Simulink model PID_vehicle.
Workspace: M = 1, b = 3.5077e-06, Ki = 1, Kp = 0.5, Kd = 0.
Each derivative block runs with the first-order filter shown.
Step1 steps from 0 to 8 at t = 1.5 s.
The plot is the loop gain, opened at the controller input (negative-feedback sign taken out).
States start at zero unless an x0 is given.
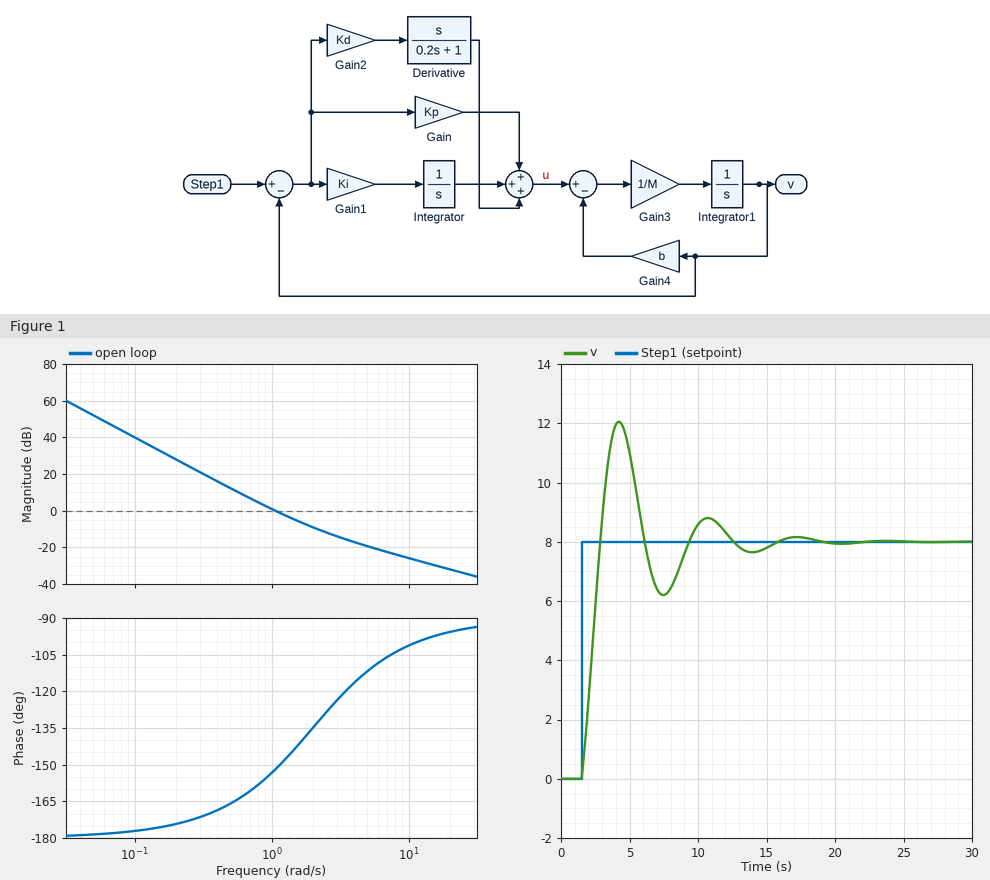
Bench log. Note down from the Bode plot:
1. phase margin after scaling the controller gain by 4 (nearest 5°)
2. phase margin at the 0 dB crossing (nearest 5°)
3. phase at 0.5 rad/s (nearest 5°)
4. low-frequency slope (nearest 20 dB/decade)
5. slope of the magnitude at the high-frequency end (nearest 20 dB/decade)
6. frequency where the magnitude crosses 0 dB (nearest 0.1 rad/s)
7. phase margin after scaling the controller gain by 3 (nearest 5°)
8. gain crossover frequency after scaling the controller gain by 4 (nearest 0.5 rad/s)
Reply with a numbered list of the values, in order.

1. 50°
2. 30°
3. -165°
4. -40 dB/decade
5. -20 dB/decade
6. 1.1 rad/s
7. 45°
8. 2.5 rad/s
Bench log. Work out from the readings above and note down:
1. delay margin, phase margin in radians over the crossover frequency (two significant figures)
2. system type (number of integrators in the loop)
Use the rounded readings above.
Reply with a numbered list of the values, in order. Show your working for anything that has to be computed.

1. 30 × π / 180 / 1.1 = 0.48 s
2. 2
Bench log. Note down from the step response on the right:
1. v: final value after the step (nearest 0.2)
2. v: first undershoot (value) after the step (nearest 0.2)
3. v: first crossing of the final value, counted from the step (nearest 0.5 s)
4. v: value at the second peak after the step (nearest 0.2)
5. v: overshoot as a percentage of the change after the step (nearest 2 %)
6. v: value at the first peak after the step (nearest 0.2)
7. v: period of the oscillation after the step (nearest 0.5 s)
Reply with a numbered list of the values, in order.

1. 8.0
2. 6.2
3. 1.5 s
4. 8.8
5. 50 %
6. 12.0
7. 6.5 s
